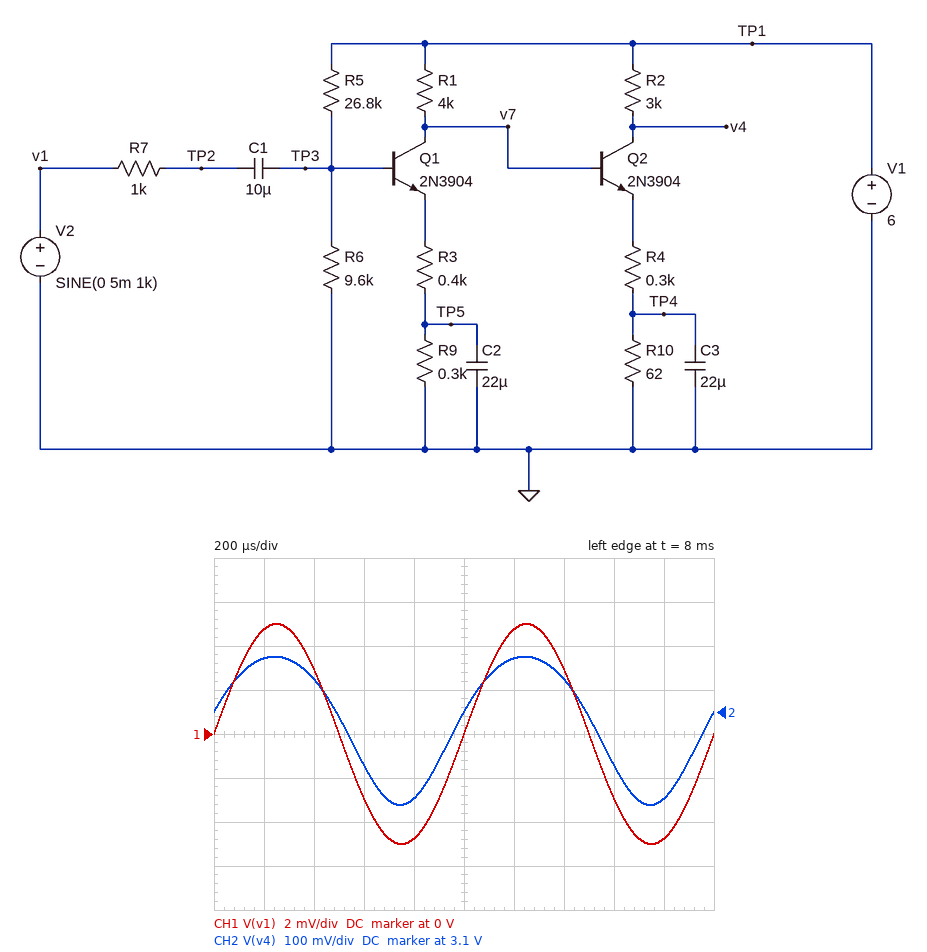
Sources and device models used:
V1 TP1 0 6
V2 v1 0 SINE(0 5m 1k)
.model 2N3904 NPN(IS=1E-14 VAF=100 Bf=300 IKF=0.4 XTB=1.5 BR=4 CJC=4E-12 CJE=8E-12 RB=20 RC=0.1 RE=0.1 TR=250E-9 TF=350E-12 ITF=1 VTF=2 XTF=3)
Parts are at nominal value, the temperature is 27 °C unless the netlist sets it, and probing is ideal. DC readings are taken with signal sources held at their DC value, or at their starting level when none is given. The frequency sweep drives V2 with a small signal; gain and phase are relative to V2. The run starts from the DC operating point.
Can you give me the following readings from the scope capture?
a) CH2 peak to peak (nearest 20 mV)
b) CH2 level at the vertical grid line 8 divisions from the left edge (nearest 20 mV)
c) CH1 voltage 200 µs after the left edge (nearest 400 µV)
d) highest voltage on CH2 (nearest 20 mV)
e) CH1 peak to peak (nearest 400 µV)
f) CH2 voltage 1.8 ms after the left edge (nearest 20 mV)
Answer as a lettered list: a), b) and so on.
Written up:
a) 340 mV
b) 2.98 V
c) 4.8 mV
d) 3.22 V
e) 10.0 mV
f) 2.90 V
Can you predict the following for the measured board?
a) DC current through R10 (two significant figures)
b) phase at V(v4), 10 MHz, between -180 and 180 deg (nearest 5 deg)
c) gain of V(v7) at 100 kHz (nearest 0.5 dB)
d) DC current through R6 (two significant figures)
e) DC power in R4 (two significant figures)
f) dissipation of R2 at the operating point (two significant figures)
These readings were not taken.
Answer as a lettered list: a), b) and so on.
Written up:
a) 970 µA
b) 155 deg
c) 10.5 dB
d) 160 µA
e) 280 µW
f) 2.8 mW
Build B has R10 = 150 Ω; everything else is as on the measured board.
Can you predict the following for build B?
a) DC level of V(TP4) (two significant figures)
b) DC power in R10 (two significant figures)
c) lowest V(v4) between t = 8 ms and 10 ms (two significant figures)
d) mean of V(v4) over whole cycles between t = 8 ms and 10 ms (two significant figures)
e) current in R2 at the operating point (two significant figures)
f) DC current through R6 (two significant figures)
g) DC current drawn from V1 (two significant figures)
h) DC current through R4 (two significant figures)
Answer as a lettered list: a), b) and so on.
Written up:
a) 120 mV
b) 95 µW
c) 3.4 V
d) 3.6 V
e) 790 µA
f) 160 µA
g) 2.2 mA
h) 800 µA
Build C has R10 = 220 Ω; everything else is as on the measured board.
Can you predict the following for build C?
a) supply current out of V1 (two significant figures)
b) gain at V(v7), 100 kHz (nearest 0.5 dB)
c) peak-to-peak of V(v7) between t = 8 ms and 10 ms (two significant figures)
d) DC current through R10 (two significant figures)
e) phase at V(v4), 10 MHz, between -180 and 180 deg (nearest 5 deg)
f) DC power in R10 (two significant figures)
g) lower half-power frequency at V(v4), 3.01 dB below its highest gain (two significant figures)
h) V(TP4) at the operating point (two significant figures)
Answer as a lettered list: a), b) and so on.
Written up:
a) 2.1 mA
b) 10.5 dB
c) 38 mV
d) 700 µA
e) 160 deg
f) 110 µW
g) 48 Hz
h) 150 mV
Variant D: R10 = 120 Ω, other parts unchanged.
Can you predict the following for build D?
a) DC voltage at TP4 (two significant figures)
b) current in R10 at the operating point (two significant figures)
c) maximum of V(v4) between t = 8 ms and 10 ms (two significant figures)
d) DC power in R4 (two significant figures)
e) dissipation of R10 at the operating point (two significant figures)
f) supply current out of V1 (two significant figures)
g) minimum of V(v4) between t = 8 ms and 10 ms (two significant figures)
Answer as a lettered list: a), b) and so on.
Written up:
a) 100 mV
b) 850 µA
c) 3.6 V
d) 220 µW
e) 86 µW
f) 2.3 mA
g) 3.3 V
